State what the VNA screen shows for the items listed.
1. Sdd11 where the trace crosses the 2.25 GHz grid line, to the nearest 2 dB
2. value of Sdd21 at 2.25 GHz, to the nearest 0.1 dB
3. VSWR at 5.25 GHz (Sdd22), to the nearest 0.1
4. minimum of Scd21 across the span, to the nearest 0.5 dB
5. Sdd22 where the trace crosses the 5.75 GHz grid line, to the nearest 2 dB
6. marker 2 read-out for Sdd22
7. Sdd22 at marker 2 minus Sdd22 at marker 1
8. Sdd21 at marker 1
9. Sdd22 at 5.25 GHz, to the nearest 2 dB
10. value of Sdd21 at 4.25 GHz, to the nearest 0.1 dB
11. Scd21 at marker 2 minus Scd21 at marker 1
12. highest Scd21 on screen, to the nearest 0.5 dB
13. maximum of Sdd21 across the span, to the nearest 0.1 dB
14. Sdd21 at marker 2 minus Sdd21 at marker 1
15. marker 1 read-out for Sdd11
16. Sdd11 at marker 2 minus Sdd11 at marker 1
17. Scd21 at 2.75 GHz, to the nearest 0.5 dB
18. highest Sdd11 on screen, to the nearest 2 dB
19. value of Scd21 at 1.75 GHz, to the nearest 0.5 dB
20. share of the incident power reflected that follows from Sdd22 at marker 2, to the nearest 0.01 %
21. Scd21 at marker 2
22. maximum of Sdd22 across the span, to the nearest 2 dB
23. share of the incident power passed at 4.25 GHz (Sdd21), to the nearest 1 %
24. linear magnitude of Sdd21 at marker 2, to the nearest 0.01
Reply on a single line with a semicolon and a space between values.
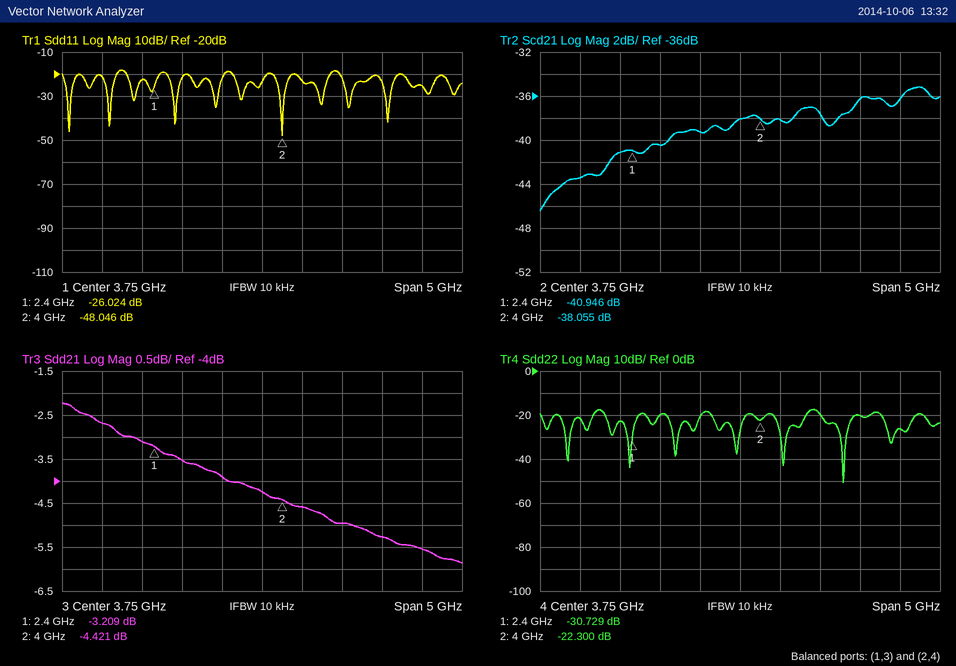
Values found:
-22 dB; -3.1 dB; 1.2; -46.5 dB; -26 dB; -22.300 dB; 8.429 dB; -3.209 dB; -20 dB; -4.6 dB; 2.891 dB; -35.0 dB; -2.2 dB; -1.212 dB; -26.024 dB; -22.022 dB; -40.5 dB; -18 dB; -43.5 dB; 0.59 %; -38.055 dB; -18 dB; 35 %; 0.60
